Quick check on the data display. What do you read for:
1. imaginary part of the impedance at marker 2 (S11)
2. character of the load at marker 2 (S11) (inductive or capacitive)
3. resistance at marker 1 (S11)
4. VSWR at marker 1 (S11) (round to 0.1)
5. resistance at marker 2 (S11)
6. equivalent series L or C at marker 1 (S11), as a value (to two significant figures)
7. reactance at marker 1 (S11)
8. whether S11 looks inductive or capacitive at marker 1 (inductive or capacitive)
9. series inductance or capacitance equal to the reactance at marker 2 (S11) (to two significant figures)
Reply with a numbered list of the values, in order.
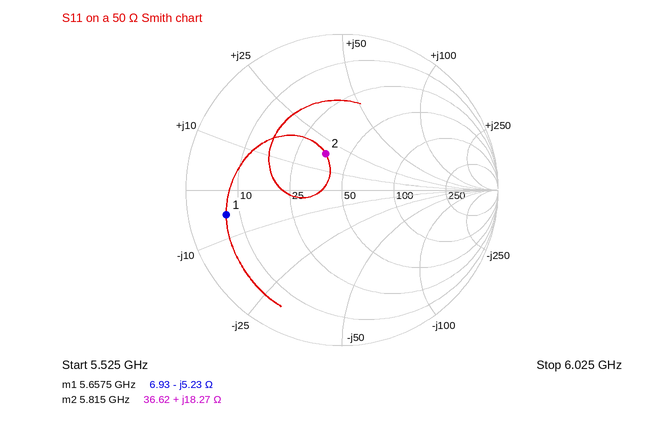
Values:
1. +18.27 Ω
2. inductive
3. 6.93 Ω
4. 7.3
5. 36.62 Ω
6. 5.4 pF
7. -5.23 Ω
8. capacitive
9. 500 pH
